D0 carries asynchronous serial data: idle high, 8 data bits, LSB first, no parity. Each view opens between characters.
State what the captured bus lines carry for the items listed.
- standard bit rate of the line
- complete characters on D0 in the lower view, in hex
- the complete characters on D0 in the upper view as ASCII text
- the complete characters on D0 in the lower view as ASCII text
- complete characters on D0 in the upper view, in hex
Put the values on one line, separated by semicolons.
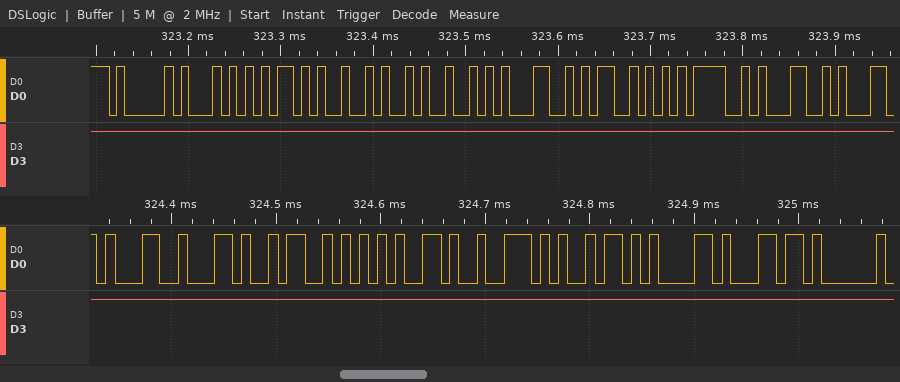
115200 baud; 31, 2C, 53, 65, 72, 69, 61, 6C; "AT+JRLS=1"; "1,Serial"; 41, 54, 2B, 4A, 52, 4C, 53, 3D, 31
